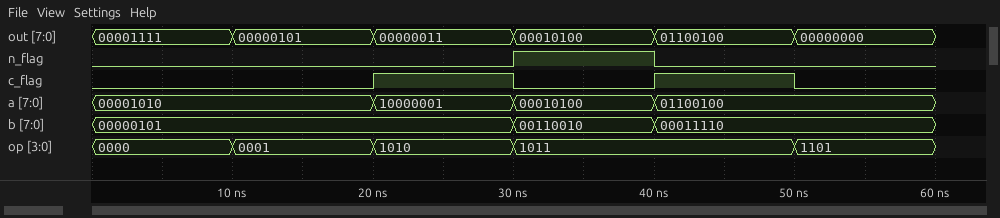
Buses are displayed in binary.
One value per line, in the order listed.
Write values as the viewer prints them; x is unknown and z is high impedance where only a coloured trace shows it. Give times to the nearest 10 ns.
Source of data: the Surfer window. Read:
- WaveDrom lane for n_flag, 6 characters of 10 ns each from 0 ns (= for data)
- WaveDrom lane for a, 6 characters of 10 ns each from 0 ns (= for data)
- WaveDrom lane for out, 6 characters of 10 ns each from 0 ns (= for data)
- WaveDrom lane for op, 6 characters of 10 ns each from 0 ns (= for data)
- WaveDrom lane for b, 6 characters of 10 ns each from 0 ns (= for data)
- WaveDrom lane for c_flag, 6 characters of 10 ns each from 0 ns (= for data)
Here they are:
{name: 'n_flag', wave: '0..10.'}
{name: 'a', wave: '=.===.', data: '00001010 10000001 00010100 01100100'}
{name: 'out', wave: '======', data: '00001111 00000101 00000011 00010100 01100100 00000000'}
{name: 'op', wave: '====.=', data: '0000 0001 1010 1011 1101'}
{name: 'b', wave: '=..==.', data: '00000101 00110010 00011110'}
{name: 'c_flag', wave: '0.1010'}
